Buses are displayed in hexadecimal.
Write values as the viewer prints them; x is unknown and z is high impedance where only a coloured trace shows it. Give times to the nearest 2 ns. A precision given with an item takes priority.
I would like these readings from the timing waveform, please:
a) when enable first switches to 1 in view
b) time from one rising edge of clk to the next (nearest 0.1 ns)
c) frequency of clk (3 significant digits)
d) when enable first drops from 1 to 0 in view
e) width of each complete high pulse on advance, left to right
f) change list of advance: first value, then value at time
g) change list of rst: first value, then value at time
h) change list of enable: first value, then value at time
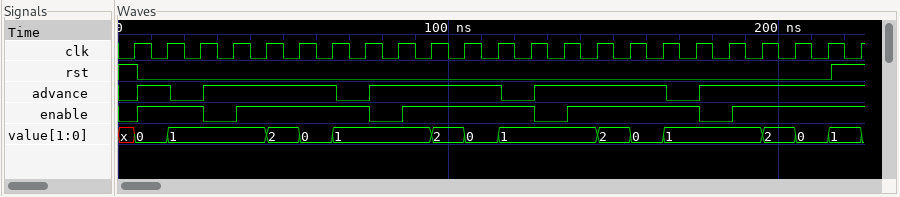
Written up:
6 ns
10 ns
100 MHz
26 ns
10 ns, 40 ns, 40 ns, 40 ns
0, 1 at 6 ns, 0 at 16 ns, 1 at 26 ns, 0 at 66 ns, 1 at 76 ns, 0 at 116 ns, 1 at 126 ns, 0 at 166 ns, 1 at 176 ns
1, 0 at 6 ns, 1 at 216 ns
0, 1 at 6 ns, 0 at 26 ns, 1 at 36 ns, 0 at 76 ns, 1 at 86 ns, 0 at 126 ns, 1 at 136 ns, 0 at 176 ns, 1 at 186 ns
